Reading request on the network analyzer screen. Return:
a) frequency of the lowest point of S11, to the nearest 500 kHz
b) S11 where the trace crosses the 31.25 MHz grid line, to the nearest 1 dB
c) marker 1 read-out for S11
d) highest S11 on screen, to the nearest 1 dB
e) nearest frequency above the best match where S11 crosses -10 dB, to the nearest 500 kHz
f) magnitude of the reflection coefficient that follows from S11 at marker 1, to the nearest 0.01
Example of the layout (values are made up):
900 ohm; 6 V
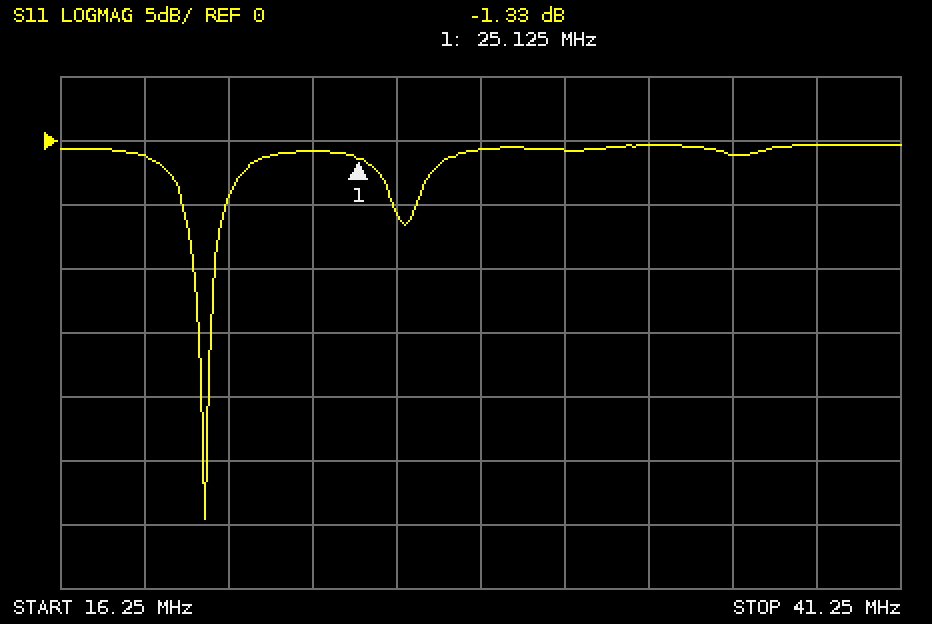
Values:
20.5 MHz; -1 dB; -1.33 dB; 0 dB; 21.0 MHz; 0.86
